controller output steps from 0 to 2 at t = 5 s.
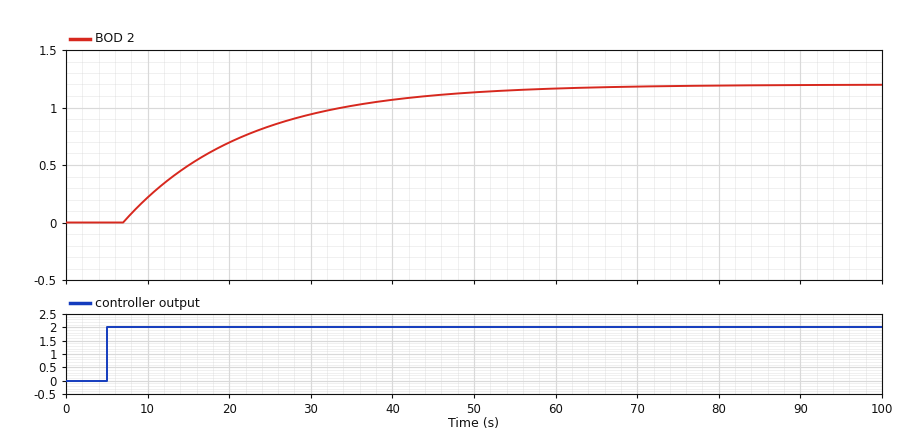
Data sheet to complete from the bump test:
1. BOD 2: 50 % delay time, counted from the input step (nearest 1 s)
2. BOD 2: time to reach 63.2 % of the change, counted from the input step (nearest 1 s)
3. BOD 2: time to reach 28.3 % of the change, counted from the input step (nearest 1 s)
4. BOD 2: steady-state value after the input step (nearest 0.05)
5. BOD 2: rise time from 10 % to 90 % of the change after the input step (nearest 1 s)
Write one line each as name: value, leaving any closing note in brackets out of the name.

BOD 2: 50 % delay time, counted from the input step: 12 s
BOD 2: time to reach 63.2 % of the change, counted from the input step: 17 s
BOD 2: time to reach 28.3 % of the change, counted from the input step: 7 s
BOD 2: steady-state value after the input step: 1.20
BOD 2: rise time from 10 % to 90 % of the change after the input step: 33 s
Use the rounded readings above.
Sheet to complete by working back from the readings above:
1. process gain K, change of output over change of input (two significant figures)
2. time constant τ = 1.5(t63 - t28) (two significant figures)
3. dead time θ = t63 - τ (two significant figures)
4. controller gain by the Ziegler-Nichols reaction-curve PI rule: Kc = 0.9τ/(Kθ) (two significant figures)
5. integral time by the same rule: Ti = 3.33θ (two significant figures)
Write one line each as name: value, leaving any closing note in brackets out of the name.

process gain K, change of output over change of input: 0.60
time constant τ = 1.5(t63 - t28): 15 s
dead time θ = t63 - τ: 2.0 s
controller gain by the Ziegler-Nichols reaction-curve PI rule: Kc = 0.9τ/(Kθ): 11
integral time by the same rule: Ti = 3.33θ: 6.7 s
